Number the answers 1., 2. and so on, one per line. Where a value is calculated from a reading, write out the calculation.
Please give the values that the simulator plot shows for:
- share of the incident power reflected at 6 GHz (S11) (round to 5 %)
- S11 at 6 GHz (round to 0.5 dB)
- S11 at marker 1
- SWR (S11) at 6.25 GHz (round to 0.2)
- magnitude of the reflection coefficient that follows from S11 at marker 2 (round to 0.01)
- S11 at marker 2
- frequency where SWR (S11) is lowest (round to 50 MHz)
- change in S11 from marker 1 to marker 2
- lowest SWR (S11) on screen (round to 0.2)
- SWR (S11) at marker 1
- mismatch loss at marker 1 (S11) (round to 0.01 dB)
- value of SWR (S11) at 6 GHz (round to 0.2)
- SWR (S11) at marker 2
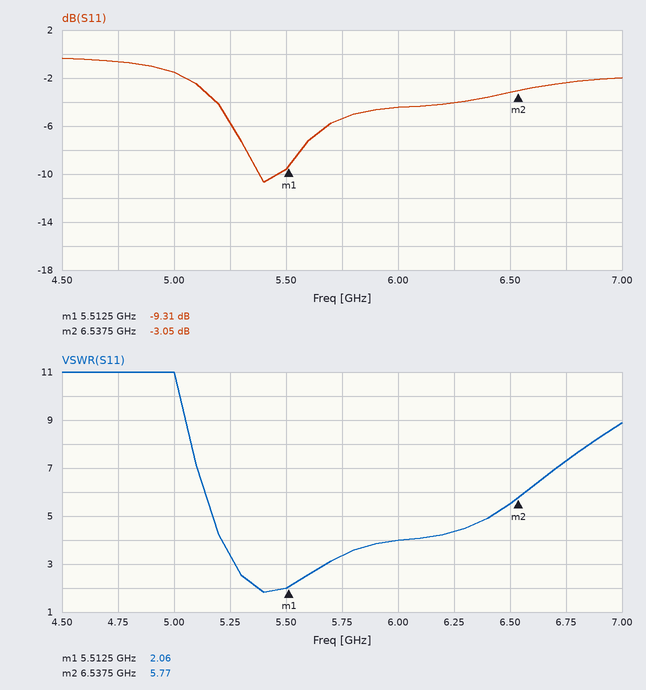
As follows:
1. 10^(-4.5/10) ≈ 35 %
2. -4.5 dB
3. -9.31 dB
4. 4.4
5. 10^(-3.05/20) ≈ 0.70
6. -3.05 dB
7. 5.40 GHz
8. -3.05 − (-9.31) = 6.26 dB
9. 1.8
10. 2.06
11. −10 log10(1 − 10^(-9.31/10)) ≈ 0.54 dB
12. 4.0
13. 5.77
